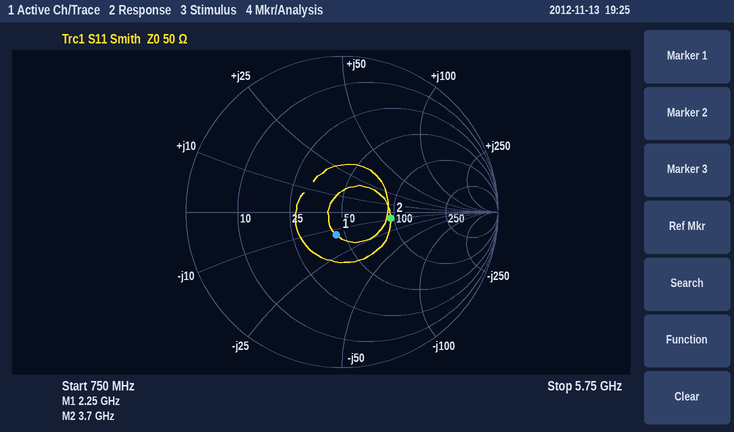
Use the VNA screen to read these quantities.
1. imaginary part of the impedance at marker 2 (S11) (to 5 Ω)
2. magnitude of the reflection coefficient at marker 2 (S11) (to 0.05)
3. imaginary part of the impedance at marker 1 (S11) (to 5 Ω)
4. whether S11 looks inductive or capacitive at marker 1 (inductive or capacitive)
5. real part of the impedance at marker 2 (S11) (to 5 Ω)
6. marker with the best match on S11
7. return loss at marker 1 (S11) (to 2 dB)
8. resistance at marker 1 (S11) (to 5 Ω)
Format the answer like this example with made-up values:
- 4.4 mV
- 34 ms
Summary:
- -10 Ω
- 0.30
- -15 Ω
- capacitive
- 95 Ω
- marker 1
- 16 dB
- 45 Ω
